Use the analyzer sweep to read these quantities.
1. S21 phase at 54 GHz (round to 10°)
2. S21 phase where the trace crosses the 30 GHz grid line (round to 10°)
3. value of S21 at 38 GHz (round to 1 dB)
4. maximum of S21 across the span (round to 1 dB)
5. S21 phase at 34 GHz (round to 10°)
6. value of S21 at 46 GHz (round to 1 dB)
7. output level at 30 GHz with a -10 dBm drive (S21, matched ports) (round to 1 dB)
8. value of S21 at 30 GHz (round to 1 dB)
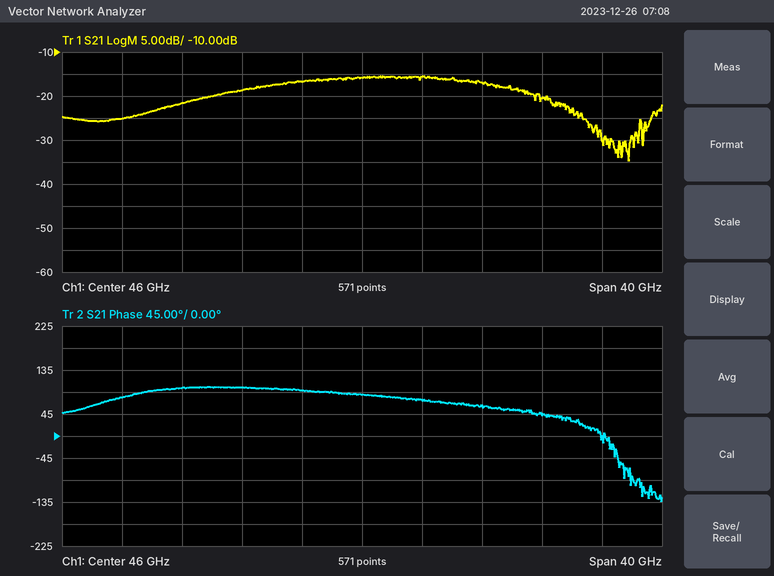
60°
80°
-19 dB
-15 dB
100°
-16 dB
-35 dBm
-25 dB
